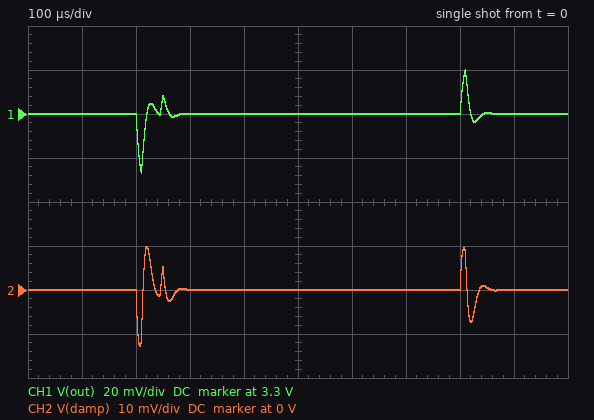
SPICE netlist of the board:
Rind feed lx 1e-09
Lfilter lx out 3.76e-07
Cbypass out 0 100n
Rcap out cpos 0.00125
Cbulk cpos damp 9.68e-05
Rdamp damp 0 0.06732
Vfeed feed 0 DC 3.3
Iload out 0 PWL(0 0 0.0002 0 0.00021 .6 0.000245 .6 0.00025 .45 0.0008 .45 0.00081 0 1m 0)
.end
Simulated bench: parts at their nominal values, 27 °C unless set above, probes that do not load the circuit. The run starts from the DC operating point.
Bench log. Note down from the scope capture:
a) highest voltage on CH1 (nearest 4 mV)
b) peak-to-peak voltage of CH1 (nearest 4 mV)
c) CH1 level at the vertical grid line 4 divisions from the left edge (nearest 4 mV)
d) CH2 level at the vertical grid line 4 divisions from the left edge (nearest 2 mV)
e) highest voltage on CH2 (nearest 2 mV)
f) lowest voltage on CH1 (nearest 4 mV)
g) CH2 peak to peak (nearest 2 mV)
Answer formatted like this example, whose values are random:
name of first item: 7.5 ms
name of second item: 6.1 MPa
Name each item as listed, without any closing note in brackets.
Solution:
highest voltage on CH1: 3.320 V
peak-to-peak voltage of CH1: 48 mV
CH1 level at the vertical grid line 4 divisions from the left edge: 3.300 V
CH2 level at the vertical grid line 4 divisions from the left edge: 0 V
highest voltage on CH2: 10 mV
lowest voltage on CH1: 3.272 V
CH2 peak to peak: 22 mV
